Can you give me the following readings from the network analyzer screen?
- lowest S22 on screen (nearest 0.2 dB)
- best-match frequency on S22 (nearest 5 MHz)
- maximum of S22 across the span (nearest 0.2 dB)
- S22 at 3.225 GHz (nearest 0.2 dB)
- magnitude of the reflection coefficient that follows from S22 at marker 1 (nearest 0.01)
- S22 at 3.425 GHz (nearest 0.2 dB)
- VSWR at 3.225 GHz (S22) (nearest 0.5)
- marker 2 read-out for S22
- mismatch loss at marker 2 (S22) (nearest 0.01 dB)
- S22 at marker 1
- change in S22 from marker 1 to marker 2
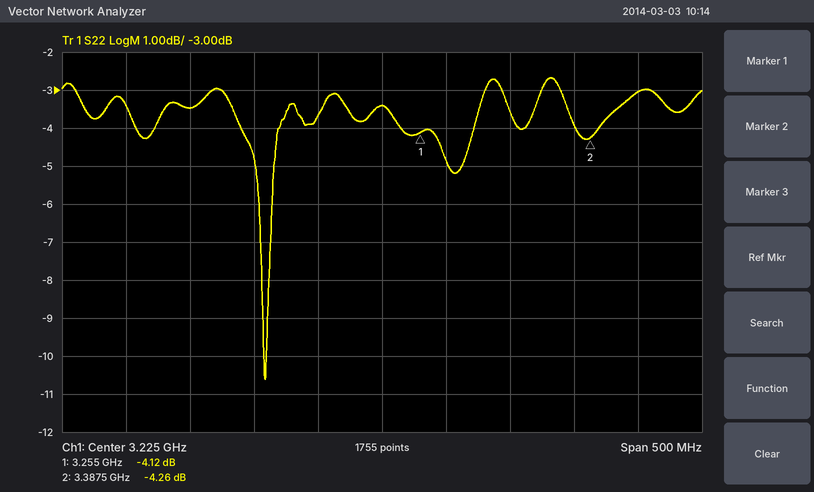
-10.6 dB
3.135 GHz
-2.6 dB
-3.4 dB
0.62
-3.0 dB
5.0
-4.26 dB
2.04 dB
-4.12 dB
-0.14 dB
